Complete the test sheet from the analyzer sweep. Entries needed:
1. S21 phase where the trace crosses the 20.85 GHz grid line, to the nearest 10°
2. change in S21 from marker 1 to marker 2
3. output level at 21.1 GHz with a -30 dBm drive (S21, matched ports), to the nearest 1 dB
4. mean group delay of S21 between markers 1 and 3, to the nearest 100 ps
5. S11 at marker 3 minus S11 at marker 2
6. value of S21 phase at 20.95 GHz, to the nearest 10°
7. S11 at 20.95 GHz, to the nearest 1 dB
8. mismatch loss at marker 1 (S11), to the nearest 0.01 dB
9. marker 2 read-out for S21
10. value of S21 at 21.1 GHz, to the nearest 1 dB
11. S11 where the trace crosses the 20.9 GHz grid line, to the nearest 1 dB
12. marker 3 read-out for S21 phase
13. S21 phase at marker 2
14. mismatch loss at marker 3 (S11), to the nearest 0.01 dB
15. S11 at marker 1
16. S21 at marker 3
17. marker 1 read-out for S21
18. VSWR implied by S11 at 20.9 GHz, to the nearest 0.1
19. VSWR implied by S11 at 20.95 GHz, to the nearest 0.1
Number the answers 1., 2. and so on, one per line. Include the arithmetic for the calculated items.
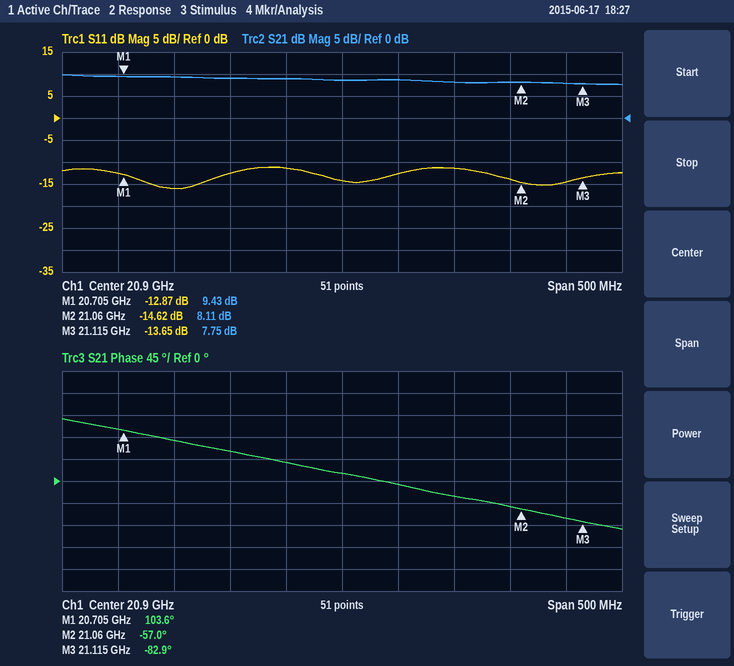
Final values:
1. 40°
2. 8.11 − (9.43) = -1.32 dB
3. -30 dBm + (8 dB) = -22 dBm
4. −(-82.9° − (103.6°))/(360° × 410 MHz) ≈ 1.3 ns
5. -13.65 − (-14.62) = 0.97 dB
6. -10°
7. -13 dB
8. −10 log10(1 − 10^(-12.87/10)) ≈ 0.23 dB
9. 8.11 dB
10. 8 dB
11. -14 dB
12. -82.9°
13. -57.0°
14. −10 log10(1 − 10^(-13.65/10)) ≈ 0.19 dB
15. -12.87 dB
16. 7.75 dB
17. 9.43 dB
18. |Γ| = 10^(-14/20) = 0.1995; VSWR = (1 + 0.1995)/(1 − 0.1995) ≈ 1.5
19. |Γ| = 10^(-13/20) = 0.2239; VSWR = (1 + 0.2239)/(1 − 0.2239) ≈ 1.6
